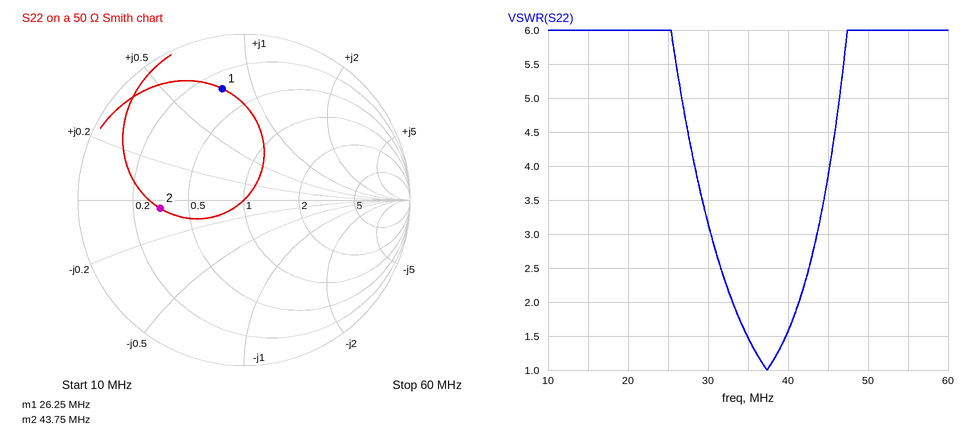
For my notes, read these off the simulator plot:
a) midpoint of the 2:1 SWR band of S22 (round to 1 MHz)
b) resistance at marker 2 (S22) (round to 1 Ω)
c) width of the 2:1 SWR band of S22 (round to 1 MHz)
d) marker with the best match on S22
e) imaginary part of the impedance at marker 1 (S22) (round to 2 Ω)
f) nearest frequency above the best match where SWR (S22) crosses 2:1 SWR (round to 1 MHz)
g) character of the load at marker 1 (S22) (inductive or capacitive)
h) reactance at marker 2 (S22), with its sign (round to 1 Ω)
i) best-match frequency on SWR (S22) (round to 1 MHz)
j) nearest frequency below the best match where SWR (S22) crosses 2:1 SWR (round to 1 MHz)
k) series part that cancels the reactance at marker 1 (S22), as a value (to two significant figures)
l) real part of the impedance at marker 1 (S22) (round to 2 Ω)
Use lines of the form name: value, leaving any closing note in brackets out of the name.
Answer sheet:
midpoint of the 2:1 SWR band of S22: 37 MHz
resistance at marker 2 (S22): 16 Ω
width of the 2:1 SWR band of S22: 8 MHz
marker with the best match on S22: marker 2
imaginary part of the impedance at marker 1 (S22): +38 Ω
nearest frequency above the best match where SWR (S22) crosses 2:1 SWR: 41 MHz
character of the load at marker 1 (S22): inductive
reactance at marker 2 (S22), with its sign: -2 Ω
best-match frequency on SWR (S22): 37 MHz
nearest frequency below the best match where SWR (S22) crosses 2:1 SWR: 33 MHz
series part that cancels the reactance at marker 1 (S22), as a value: 160 pF
real part of the impedance at marker 1 (S22): 16 Ω
